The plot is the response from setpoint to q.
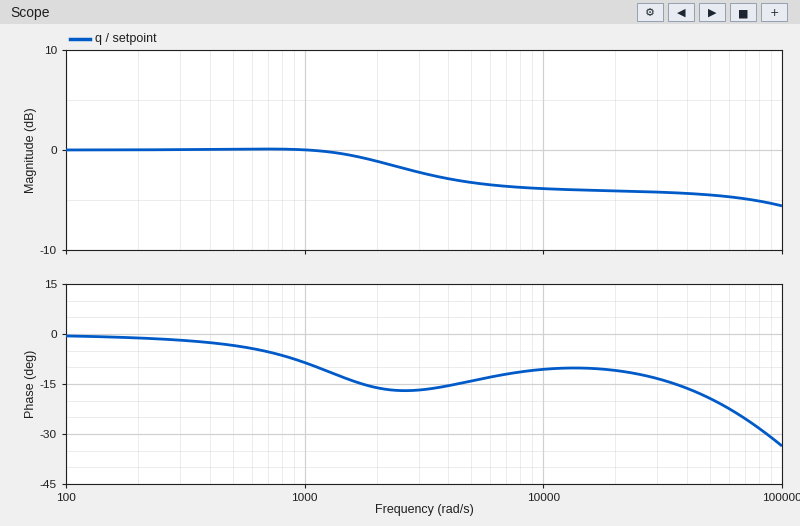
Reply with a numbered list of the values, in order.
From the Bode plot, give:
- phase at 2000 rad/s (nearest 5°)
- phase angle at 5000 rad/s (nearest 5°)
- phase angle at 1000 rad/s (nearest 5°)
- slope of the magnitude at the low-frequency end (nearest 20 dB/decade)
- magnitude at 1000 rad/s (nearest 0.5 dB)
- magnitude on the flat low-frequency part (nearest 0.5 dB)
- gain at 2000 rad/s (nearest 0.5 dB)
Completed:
1. -15°
2. -15°
3. -10°
4. 0 dB/decade
5. 0.0 dB
6. 0.0 dB
7. -1.0 dB
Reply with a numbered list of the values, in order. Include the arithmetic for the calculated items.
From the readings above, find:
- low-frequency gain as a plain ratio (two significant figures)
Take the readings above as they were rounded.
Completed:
1. 10^(0 / 20) = 1.0
